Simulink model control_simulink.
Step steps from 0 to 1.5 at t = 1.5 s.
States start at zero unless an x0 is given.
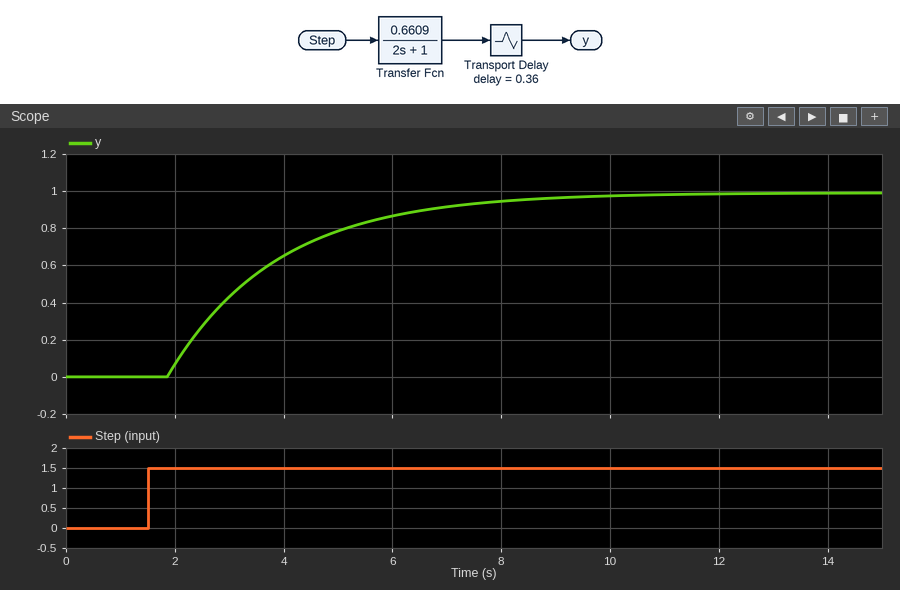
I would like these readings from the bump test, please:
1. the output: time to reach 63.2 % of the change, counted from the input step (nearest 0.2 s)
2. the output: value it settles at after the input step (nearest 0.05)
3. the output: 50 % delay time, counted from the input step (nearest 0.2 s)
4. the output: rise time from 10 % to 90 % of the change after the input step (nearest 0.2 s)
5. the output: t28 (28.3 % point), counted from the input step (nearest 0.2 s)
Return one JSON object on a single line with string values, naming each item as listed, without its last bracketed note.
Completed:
{"the output: time to reach 63.2 % of the change, counted from the input step": "2.4 s", "the output: value it settles at after the input step": "1.00", "the output: 50 % delay time, counted from the input step": "1.8 s", "the output: rise time from 10 % to 90 % of the change after the input step": "4.4 s", "the output: t28 (28.3 % point), counted from the input step": "1.0 s"}
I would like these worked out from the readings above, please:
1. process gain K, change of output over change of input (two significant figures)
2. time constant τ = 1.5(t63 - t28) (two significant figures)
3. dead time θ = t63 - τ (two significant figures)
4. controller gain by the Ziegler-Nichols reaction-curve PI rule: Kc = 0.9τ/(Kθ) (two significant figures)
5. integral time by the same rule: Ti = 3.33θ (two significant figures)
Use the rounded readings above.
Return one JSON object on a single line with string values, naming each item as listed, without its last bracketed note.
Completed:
{"process gain K, change of output over change of input": "0.67", "time constant τ = 1.5(t63 - t28)": "2.1 s", "dead time θ = t63 - τ": "0.30 s", "controller gain by the Ziegler-Nichols reaction-curve PI rule: Kc = 0.9τ/(Kθ)": "9.4", "integral time by the same rule: Ti = 3.33θ": "1.00 s"}
